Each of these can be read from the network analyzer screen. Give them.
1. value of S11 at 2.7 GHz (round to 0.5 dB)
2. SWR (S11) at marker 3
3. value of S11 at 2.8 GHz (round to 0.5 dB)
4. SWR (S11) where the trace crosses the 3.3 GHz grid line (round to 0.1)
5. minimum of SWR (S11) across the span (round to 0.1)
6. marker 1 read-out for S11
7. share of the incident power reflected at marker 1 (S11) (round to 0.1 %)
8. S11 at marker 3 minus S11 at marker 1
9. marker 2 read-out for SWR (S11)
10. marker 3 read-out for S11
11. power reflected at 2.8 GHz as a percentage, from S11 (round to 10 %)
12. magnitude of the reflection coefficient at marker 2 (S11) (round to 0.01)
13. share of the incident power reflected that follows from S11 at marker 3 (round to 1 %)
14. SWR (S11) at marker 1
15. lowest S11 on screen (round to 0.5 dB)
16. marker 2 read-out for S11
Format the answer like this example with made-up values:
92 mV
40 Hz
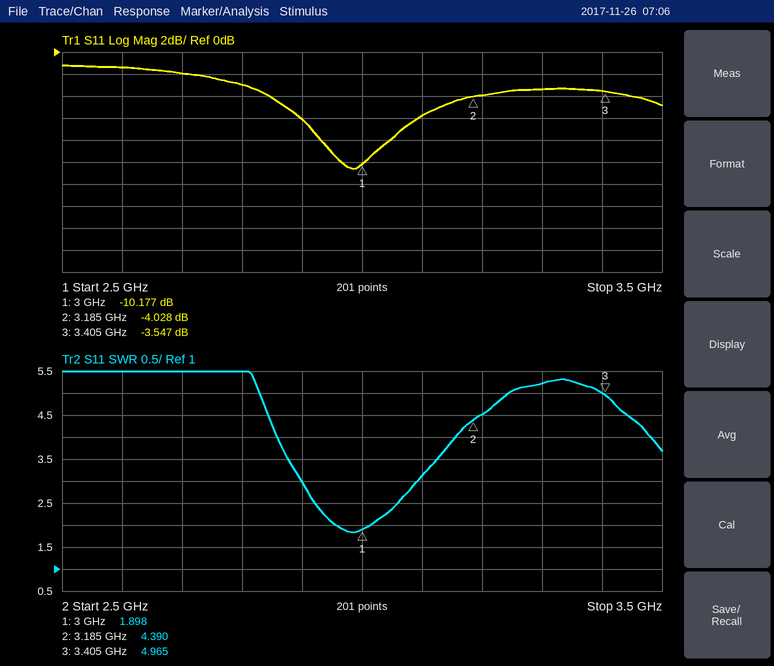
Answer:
-2.0 dB
4.965
-3.0 dB
5.2
1.8
-10.177 dB
9.6 %
6.630 dB
4.390
-3.547 dB
50 %
0.63
44 %
1.898
-10.5 dB
-4.028 dB
